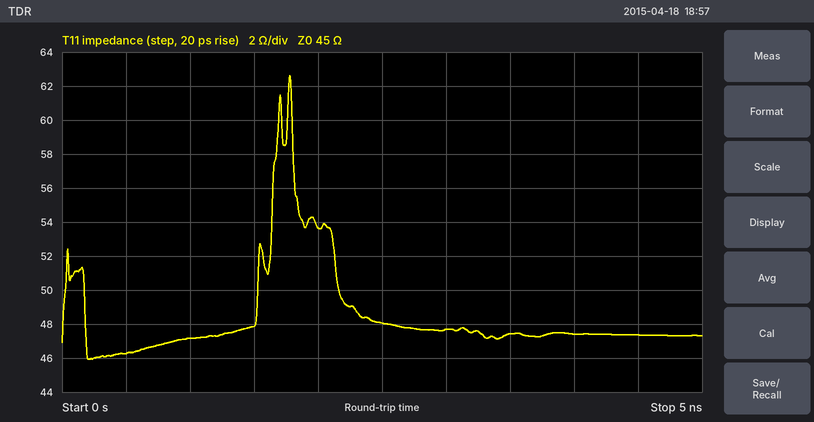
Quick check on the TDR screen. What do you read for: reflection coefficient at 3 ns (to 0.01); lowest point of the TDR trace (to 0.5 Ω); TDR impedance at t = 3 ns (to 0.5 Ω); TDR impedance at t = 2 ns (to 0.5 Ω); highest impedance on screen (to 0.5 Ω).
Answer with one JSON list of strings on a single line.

["+0.03", "46.0 Ω", "47.5 Ω", "53.5 Ω", "62.5 Ω"]
